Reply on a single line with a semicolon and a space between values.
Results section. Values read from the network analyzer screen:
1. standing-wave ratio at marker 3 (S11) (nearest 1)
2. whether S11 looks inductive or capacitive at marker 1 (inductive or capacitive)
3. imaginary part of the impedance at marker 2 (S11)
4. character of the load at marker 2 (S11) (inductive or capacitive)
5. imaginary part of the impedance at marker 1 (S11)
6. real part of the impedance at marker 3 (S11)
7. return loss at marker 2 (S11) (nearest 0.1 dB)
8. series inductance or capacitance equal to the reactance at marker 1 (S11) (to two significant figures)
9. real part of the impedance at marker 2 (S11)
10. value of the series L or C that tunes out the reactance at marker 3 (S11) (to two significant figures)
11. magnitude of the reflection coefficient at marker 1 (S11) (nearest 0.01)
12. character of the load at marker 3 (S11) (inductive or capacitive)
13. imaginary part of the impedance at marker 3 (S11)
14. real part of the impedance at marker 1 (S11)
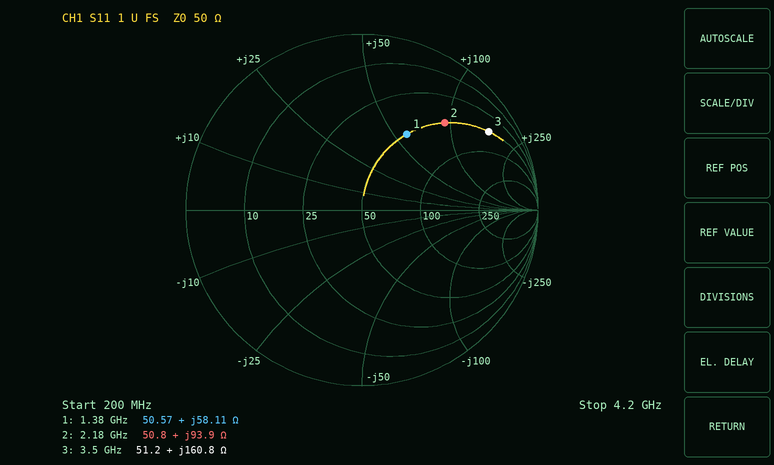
12; inductive; +93.9 Ω; inductive; +58.11 Ω; 51.2 Ω; 3.3 dB; 6.7 nH; 50.8 Ω; 280 fF; 0.50; inductive; +160.8 Ω; 50.57 Ω
